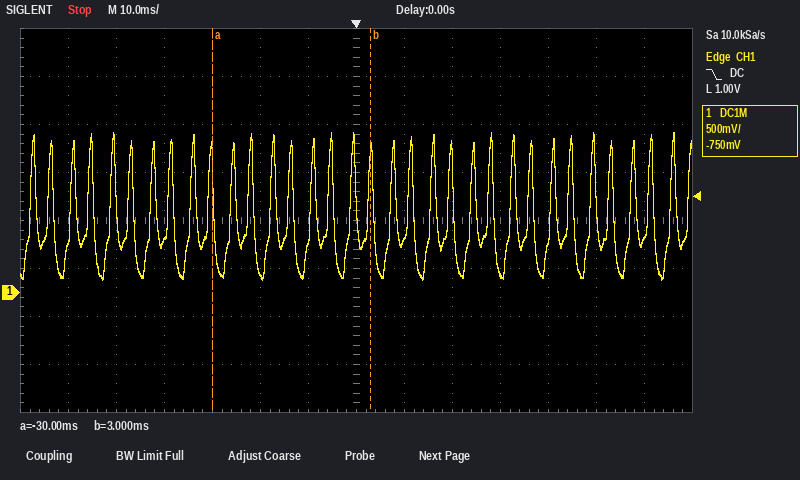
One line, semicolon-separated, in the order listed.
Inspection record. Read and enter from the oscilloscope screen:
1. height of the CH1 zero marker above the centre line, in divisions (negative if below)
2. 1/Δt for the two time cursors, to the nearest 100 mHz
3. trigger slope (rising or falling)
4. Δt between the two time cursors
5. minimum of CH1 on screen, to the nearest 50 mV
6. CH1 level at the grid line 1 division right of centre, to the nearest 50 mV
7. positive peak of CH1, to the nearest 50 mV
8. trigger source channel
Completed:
-1.5 div; 30.3 Hz; falling; 33 ms; 150 mV; 550 mV; 1.65 V; CH1
